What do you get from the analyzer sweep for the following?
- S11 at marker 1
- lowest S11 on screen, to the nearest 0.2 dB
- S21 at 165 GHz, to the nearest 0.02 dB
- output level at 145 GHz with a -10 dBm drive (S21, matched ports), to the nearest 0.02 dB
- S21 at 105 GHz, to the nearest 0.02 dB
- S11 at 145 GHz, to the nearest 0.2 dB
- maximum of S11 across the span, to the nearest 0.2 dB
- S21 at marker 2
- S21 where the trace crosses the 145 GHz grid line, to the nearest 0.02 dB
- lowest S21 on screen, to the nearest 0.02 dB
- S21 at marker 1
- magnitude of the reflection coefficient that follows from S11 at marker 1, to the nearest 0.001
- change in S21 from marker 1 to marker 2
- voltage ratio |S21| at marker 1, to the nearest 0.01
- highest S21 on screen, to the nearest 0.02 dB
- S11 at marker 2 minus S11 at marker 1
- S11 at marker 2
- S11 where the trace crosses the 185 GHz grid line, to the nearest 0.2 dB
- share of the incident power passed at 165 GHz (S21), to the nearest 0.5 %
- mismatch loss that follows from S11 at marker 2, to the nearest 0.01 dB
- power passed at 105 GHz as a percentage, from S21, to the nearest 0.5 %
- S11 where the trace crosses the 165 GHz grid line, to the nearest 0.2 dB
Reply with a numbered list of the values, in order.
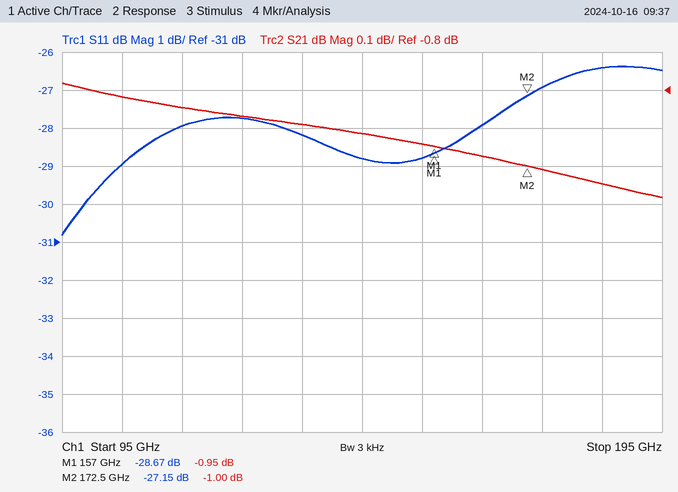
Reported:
1. -28.67 dB
2. -30.8 dB
3. -0.98 dB
4. -10.92 dBm
5. -0.82 dB
6. -28.8 dB
7. -26.4 dB
8. -1.00 dB
9. -0.92 dB
10. -1.08 dB
11. -0.95 dB
12. 0.037
13. -0.05 dB
14. 0.90
15. -0.78 dB
16. 1.52 dB
17. -27.15 dB
18. -26.4 dB
19. 80.0 %
20. 0.01 dB
21. 83.0 %
22. -28.0 dB
